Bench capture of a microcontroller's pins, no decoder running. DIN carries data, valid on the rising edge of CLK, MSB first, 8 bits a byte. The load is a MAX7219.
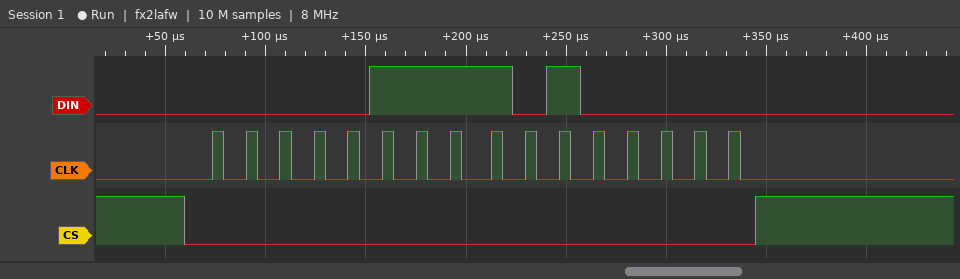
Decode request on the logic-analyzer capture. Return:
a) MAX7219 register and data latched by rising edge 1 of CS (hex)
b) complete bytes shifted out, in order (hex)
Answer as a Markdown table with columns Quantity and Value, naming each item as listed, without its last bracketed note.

| Quantity | Value |
|---|---|
| MAX7219 register and data latched by rising edge 1 of CS | register 0x7, data 0xA0 |
| complete bytes shifted out, in order | 07 A0 |
